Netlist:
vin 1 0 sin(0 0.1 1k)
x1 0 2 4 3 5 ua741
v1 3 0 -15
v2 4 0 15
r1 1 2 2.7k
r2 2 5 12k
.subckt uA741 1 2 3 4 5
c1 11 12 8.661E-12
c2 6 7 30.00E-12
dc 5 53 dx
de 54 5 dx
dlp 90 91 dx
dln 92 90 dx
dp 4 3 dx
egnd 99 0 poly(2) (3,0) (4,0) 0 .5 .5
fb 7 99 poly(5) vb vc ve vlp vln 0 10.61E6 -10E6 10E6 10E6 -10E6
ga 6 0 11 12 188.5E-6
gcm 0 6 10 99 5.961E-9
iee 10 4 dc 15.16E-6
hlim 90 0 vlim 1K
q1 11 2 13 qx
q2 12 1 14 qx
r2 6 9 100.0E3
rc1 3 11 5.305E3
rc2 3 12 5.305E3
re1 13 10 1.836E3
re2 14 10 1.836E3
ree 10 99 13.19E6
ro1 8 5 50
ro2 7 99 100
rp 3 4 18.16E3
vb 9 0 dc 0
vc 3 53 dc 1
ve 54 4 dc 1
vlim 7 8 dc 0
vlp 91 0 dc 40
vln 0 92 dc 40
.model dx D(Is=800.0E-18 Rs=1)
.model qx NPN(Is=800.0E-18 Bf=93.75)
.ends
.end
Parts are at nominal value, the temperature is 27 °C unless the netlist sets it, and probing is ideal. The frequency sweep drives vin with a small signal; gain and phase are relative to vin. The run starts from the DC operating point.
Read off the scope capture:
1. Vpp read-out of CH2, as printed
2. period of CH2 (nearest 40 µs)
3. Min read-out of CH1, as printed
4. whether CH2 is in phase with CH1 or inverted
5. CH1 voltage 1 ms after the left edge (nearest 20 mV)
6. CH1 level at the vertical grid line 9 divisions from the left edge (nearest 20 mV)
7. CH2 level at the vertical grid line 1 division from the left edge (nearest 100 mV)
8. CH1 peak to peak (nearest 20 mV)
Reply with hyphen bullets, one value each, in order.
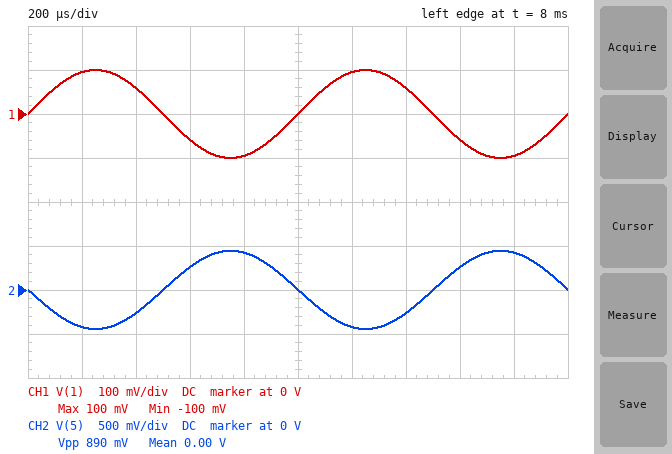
- 890 mV
- 1.00 ms
- -100 mV
- inverted
- 0 V
- -100 mV
- -400 mV
- 200 mV
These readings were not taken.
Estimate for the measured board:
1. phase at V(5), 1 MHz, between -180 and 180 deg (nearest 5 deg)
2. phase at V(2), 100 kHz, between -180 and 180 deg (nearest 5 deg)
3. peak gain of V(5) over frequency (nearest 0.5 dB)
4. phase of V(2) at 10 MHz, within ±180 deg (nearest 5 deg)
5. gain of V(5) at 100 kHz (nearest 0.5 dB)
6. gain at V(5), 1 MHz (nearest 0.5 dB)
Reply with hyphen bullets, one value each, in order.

- 70 deg
- 65 deg
- 13.0 dB
- 0 deg
- 12.0 dB
- -2.5 dB
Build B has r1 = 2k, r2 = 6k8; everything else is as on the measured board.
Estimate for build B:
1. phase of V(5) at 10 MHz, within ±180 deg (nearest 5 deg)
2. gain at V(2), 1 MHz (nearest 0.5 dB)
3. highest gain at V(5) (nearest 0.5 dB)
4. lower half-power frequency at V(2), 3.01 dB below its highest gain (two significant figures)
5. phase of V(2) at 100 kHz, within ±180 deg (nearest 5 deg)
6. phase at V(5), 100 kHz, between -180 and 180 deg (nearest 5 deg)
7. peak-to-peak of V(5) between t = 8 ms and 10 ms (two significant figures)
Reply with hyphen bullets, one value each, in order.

- 5 deg
- -1.5 dB
- 10.5 dB
- 230 kHz
- 70 deg
- 155 deg
- 680 mV
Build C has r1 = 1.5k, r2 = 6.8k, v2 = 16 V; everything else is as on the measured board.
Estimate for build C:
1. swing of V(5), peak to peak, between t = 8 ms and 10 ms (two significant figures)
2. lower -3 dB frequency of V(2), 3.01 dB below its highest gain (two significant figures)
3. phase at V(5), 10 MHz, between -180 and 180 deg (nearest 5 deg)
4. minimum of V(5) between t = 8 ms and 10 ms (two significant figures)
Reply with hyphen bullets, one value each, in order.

- 910 mV
- 180 kHz
- 5 deg
- -450 mV
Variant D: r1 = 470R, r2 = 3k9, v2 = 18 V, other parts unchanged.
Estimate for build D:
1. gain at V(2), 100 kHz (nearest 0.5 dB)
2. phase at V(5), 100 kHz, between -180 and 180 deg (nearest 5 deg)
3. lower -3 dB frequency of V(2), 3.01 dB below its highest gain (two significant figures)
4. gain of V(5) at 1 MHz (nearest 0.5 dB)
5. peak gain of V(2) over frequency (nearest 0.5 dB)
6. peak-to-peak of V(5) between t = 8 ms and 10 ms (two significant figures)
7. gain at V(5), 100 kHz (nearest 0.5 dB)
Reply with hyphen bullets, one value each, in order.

- -4.0 dB
- 135 deg
- 110 kHz
- -2.0 dB
- -0.5 dB
- 1.7 V
- 16.0 dB
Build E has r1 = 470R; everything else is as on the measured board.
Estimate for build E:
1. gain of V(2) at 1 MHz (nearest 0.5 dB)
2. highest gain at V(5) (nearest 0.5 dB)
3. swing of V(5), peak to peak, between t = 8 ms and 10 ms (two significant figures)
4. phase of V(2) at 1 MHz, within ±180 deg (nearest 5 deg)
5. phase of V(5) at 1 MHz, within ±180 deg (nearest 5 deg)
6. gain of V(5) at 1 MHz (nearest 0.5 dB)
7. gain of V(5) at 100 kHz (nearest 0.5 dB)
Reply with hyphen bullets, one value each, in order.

- 0 dB
- 28.0 dB
- 5.1 V
- 0 deg
- 60 deg
- -1.5 dB
- 19.0 dB
